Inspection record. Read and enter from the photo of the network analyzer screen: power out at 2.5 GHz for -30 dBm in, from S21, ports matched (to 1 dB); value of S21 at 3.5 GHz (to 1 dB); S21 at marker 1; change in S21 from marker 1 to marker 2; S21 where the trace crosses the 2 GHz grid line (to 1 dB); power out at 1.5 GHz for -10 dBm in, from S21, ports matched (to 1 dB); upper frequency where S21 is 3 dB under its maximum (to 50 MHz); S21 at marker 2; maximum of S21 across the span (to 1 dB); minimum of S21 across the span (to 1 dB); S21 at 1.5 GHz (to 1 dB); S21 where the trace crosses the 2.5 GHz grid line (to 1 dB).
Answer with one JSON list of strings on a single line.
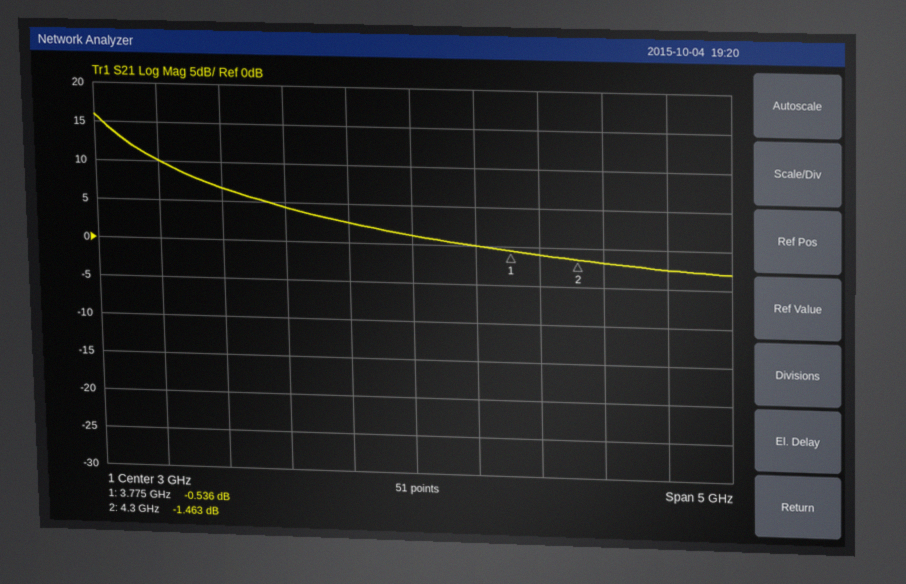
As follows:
["-27 dBm", "0 dB", "-0.536 dB", "-0.927 dB", "4 dB", "-3 dBm", "700 MHz", "-1.463 dB", "16 dB", "-3 dB", "7 dB", "3 dB"]
